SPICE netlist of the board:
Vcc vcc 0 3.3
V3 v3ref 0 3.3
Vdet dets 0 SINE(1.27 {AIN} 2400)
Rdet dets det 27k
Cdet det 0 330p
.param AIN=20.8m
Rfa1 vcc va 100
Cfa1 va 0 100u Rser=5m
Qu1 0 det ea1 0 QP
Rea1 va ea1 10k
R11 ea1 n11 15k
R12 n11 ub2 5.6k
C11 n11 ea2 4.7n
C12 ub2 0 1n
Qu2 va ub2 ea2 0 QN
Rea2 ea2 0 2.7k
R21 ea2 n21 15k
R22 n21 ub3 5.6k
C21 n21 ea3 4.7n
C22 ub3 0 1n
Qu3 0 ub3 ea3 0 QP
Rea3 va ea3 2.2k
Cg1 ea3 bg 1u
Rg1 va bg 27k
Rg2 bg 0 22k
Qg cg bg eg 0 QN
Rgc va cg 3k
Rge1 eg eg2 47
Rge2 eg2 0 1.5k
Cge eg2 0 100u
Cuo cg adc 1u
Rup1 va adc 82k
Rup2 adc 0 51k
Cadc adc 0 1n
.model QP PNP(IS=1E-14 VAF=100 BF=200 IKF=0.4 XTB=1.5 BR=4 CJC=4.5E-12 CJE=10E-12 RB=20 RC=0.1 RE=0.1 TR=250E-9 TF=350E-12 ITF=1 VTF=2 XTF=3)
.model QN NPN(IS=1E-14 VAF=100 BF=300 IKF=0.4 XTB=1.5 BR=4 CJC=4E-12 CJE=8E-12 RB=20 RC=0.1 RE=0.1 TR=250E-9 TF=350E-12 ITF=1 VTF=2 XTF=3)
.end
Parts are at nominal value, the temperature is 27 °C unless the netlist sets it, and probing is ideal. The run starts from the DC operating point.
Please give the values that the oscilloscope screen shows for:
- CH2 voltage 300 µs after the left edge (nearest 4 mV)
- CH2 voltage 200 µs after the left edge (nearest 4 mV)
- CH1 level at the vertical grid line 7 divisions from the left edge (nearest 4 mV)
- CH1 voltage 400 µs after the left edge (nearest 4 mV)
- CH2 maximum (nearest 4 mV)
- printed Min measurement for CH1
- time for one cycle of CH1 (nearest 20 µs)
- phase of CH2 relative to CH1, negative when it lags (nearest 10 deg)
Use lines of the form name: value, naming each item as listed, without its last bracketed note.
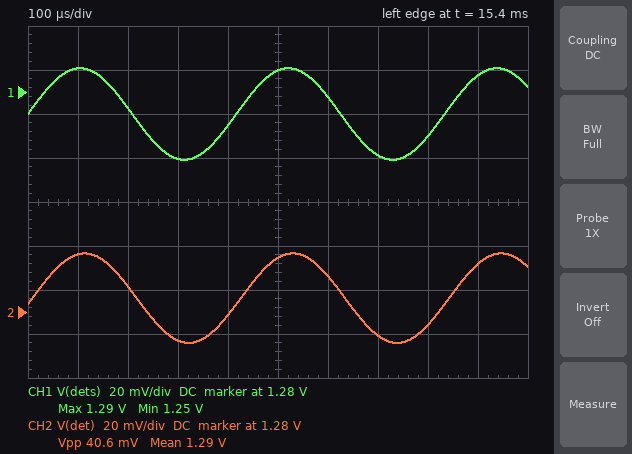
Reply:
CH2 voltage 300 µs after the left edge: 1.268 V
CH2 voltage 200 µs after the left edge: 1.292 V
CH1 level at the vertical grid line 7 divisions from the left edge: 1.252 V
CH1 voltage 400 µs after the left edge: 1.264 V
CH2 maximum: 1.308 V
printed Min measurement for CH1: 1.25 V
time for one cycle of CH1: 420 µs
phase of CH2 relative to CH1, negative when it lags: -10 deg
